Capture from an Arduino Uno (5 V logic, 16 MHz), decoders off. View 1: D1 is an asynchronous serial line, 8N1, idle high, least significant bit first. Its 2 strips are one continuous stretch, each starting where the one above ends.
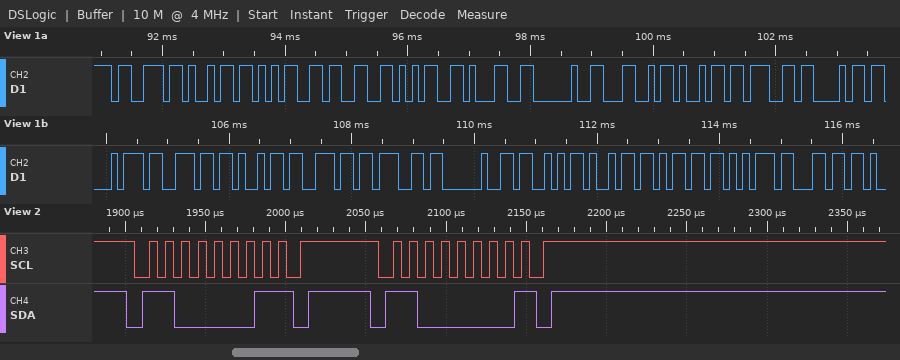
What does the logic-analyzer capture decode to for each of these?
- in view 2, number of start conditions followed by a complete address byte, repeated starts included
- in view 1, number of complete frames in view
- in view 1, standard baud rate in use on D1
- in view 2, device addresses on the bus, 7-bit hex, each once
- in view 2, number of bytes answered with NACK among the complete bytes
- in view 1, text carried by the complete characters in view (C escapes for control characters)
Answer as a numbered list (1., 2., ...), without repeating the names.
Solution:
1. 2
2. 22
3. 9600 baud
4. 0x60
5. 2
6. "si5351 Lightning Simul"
